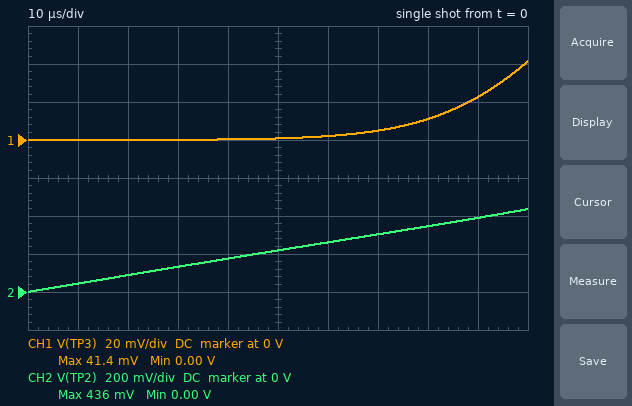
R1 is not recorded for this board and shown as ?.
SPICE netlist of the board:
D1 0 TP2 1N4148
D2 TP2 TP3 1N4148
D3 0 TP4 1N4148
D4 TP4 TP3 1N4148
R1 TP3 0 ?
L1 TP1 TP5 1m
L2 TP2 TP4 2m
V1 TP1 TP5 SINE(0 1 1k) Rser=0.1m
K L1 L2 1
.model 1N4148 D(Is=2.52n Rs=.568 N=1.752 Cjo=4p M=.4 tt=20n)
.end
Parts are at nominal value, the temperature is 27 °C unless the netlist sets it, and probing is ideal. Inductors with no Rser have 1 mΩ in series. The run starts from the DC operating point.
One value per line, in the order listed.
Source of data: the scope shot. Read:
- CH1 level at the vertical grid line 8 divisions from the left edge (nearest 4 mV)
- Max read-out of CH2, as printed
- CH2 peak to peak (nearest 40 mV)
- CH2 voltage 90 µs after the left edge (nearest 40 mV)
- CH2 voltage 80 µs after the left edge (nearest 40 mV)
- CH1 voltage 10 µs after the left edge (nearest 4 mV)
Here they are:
12 mV
436 mV
440 mV
400 mV
360 mV
0 V
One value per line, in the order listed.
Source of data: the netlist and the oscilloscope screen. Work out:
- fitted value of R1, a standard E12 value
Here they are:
2.7 kΩ
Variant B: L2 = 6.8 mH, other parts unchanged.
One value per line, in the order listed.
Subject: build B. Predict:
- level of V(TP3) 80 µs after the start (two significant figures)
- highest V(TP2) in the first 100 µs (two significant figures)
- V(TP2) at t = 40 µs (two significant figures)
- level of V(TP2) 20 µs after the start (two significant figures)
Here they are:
290 mV
1.0 V
330 mV
160 mV
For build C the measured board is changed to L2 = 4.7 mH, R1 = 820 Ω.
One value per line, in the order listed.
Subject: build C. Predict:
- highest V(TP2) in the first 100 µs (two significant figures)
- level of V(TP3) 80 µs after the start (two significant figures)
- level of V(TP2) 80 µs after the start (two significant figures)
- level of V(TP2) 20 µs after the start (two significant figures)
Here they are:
750 mV
83 mV
560 mV
140 mV
